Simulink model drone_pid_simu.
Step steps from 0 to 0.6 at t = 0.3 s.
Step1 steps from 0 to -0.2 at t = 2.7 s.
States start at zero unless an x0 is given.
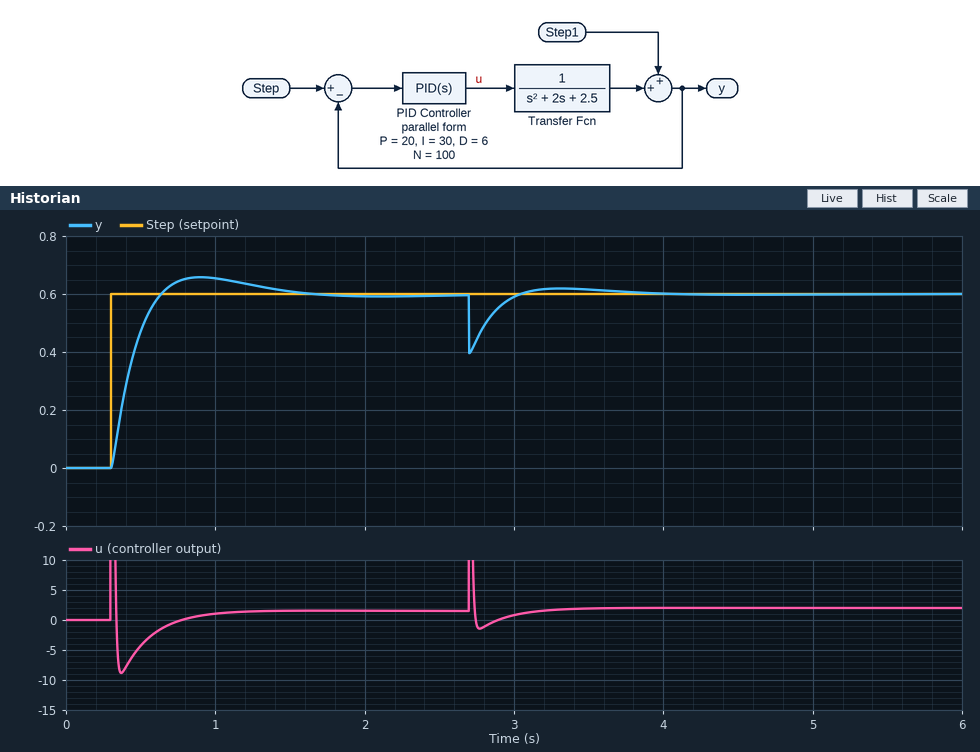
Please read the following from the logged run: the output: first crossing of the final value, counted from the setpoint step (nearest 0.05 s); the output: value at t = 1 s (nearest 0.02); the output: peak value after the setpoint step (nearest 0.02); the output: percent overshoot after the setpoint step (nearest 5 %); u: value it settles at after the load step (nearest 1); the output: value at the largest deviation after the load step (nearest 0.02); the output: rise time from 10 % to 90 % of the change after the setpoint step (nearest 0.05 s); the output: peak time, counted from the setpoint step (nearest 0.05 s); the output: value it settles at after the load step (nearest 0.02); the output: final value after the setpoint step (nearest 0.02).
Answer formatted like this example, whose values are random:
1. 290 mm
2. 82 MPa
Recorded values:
1. 0.35 s
2. 0.66
3. 0.66
4. 10 %
5. 2
6. 0.40
7. 0.25 s
8. 0.60 s
9. 0.60
10. 0.60
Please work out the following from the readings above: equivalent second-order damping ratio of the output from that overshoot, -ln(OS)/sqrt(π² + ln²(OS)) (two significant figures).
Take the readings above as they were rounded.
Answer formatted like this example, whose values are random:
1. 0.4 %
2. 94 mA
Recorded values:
1. 0.59
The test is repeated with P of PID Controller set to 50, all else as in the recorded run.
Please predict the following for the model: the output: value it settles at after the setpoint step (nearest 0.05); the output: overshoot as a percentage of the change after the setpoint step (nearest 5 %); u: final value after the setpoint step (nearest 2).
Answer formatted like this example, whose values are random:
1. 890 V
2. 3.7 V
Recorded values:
1. 0.60
2. 20 %
3. 2
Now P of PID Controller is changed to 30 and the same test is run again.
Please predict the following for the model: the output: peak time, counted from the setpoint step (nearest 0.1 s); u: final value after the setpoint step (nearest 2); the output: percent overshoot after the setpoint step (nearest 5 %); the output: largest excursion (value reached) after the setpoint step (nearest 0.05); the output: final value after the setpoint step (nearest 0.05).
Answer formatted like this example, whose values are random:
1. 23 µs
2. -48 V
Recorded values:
1. 0.5 s
2. 2
3. 15 %
4. 0.70
5. 0.60
